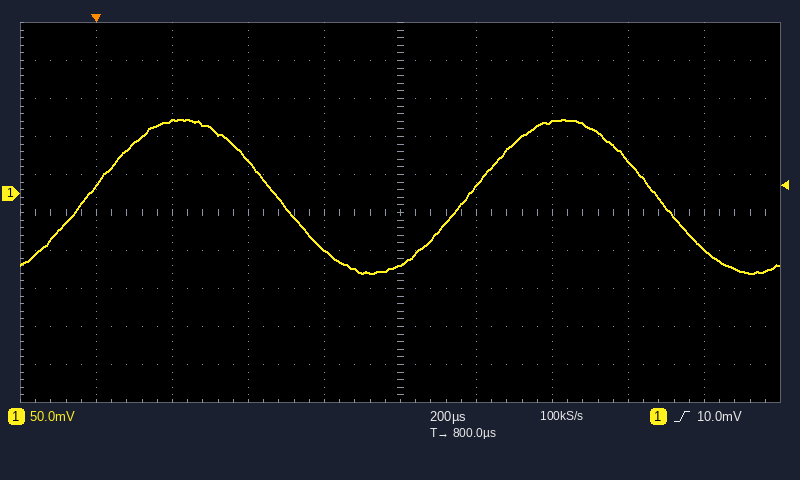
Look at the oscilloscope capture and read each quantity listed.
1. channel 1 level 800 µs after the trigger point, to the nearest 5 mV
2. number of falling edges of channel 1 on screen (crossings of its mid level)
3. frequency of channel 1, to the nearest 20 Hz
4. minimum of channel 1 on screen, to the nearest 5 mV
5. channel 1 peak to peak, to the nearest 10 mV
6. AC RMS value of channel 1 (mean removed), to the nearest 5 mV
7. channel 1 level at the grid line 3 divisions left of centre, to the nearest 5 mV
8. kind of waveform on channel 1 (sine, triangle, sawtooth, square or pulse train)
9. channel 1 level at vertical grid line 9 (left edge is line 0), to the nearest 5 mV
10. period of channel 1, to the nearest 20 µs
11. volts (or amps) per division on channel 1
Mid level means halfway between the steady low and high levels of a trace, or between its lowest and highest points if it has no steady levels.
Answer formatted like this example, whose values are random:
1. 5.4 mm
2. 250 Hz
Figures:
1. -95 mV
2. 2
3. 1.00 kHz
4. -105 mV
5. 200 mV
6. 70 mV
7. 95 mV
8. sine
9. -75 mV
10. 1.00 ms
11. 50 mV
